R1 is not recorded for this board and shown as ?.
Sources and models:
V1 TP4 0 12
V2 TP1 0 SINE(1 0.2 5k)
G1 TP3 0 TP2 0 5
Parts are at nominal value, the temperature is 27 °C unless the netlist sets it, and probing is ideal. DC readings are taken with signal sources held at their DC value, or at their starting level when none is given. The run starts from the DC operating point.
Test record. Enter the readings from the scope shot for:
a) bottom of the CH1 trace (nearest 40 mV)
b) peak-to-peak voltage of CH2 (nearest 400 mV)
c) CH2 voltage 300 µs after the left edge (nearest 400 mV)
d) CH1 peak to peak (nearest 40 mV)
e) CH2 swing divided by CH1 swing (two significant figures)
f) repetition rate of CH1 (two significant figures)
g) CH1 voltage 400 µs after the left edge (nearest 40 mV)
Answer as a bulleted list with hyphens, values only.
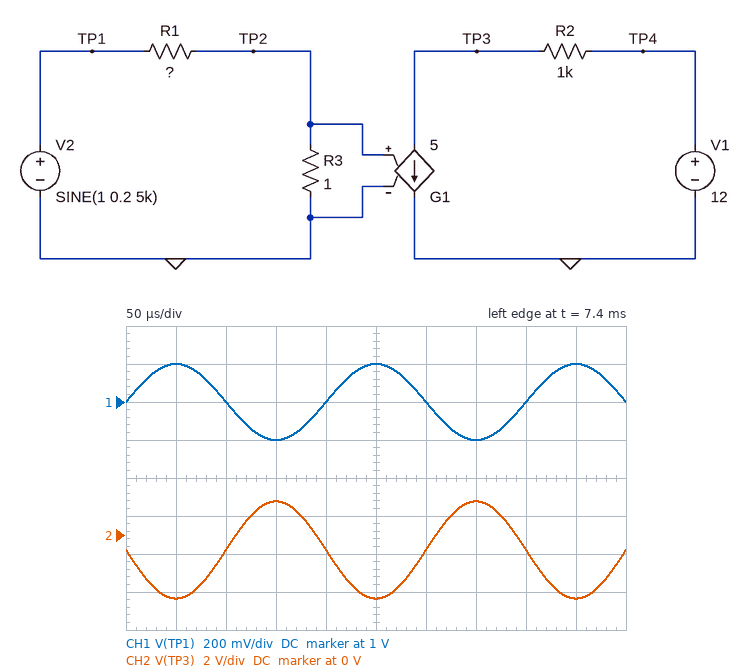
- 800 mV
- 5.2 V
- -800 mV
- 400 mV
- 13
- 5.0 kHz
- 1.00 V
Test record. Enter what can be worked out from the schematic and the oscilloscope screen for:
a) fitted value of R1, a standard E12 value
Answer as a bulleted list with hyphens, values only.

- 390 Ω
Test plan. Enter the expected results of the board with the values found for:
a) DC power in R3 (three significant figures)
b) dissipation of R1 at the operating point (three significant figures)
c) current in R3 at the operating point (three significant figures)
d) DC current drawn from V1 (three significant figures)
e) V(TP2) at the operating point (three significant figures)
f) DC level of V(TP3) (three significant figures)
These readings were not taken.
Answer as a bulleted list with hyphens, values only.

- 6.54 µW
- 2.55 mW
- 2.56 mA
- 12.8 mA
- 2.56 mV
- -788 mV
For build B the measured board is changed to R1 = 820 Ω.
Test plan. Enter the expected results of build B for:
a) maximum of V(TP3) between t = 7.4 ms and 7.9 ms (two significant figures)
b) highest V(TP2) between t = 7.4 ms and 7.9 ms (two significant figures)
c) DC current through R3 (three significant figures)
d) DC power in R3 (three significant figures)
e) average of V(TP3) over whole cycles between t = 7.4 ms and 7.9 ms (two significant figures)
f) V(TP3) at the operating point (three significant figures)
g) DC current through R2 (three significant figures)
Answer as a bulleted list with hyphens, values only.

- 7.1 V
- 1.5 mV
- 1.22 mA
- 1.48 µW
- 5.9 V
- 5.91 V
- 6.09 mA
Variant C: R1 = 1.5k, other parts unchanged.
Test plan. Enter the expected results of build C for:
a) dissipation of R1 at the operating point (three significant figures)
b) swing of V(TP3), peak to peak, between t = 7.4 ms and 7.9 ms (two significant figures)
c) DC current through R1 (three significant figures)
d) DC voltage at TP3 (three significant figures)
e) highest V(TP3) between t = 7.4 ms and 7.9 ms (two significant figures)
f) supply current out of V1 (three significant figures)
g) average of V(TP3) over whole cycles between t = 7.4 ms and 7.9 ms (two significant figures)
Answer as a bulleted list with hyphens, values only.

- 666 µW
- 1.3 V
- 666 µA
- 8.67 V
- 9.3 V
- 3.33 mA
- 8.7 V
